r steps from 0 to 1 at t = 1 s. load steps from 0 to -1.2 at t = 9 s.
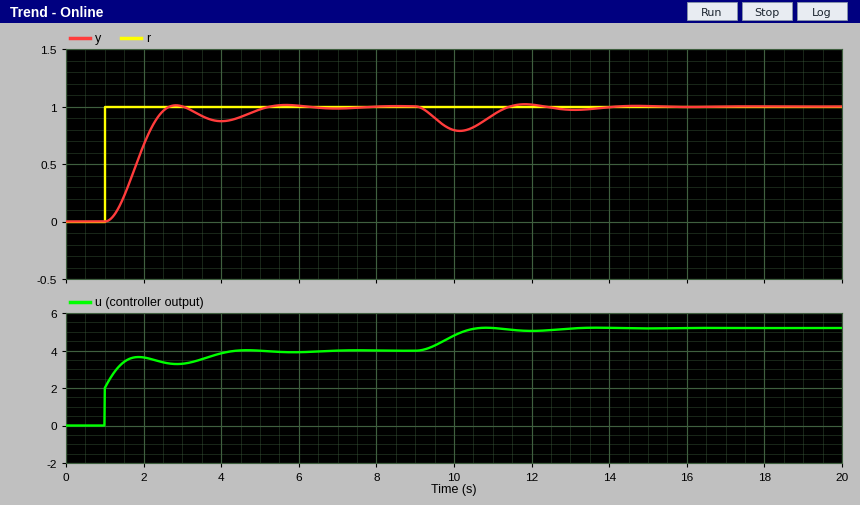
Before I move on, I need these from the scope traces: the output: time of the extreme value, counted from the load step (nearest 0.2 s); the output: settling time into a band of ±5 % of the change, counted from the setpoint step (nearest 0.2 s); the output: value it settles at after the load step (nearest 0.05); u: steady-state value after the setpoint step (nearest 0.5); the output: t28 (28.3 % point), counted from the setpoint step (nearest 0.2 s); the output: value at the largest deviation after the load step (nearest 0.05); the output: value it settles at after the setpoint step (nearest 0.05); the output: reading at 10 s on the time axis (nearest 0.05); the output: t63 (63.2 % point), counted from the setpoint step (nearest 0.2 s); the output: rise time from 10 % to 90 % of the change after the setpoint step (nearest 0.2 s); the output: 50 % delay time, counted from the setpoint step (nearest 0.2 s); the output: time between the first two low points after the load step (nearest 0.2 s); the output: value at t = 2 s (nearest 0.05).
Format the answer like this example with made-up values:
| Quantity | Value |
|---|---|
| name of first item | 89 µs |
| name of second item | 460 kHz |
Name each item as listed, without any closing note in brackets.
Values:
| Quantity | Value |
|---|---|
| the output: time of the extreme value, counted from the load step | 1.2 s |
| the output: settling time into a band of ±5 % of the change, counted from the setpoint step | 3.8 s |
| the output: value it settles at after the load step | 1.00 |
| u: steady-state value after the setpoint step | 4.0 |
| the output: t28 (28.3 % point), counted from the setpoint step | 0.6 s |
| the output: value at the largest deviation after the load step | 0.80 |
| the output: value it settles at after the setpoint step | 1.00 |
| the output: reading at 10 s on the time axis | 0.80 |
| the output: t63 (63.2 % point), counted from the setpoint step | 1.0 s |
| the output: rise time from 10 % to 90 % of the change after the setpoint step | 1.0 s |
| the output: 50 % delay time, counted from the setpoint step | 0.8 s |
| the output: time between the first two low points after the load step | 3.0 s |
| the output: value at t = 2 s | 0.65 |
